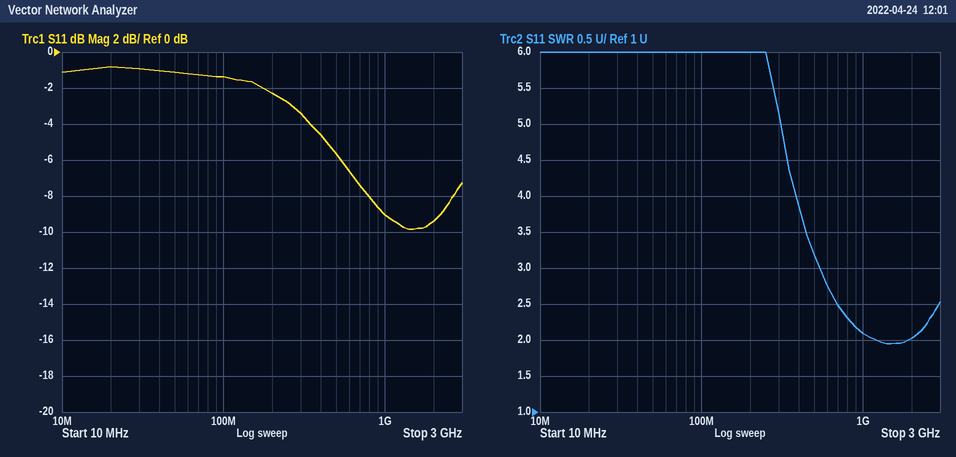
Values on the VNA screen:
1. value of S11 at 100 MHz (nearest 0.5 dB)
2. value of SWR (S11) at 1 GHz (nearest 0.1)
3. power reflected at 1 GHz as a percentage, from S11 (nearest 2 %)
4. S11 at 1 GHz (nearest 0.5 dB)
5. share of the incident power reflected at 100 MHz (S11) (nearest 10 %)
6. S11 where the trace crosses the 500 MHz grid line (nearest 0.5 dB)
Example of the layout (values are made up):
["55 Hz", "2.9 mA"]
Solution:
["-1.5 dB", "2.1", "12 %", "-9.0 dB", "70 %", "-5.5 dB"]
